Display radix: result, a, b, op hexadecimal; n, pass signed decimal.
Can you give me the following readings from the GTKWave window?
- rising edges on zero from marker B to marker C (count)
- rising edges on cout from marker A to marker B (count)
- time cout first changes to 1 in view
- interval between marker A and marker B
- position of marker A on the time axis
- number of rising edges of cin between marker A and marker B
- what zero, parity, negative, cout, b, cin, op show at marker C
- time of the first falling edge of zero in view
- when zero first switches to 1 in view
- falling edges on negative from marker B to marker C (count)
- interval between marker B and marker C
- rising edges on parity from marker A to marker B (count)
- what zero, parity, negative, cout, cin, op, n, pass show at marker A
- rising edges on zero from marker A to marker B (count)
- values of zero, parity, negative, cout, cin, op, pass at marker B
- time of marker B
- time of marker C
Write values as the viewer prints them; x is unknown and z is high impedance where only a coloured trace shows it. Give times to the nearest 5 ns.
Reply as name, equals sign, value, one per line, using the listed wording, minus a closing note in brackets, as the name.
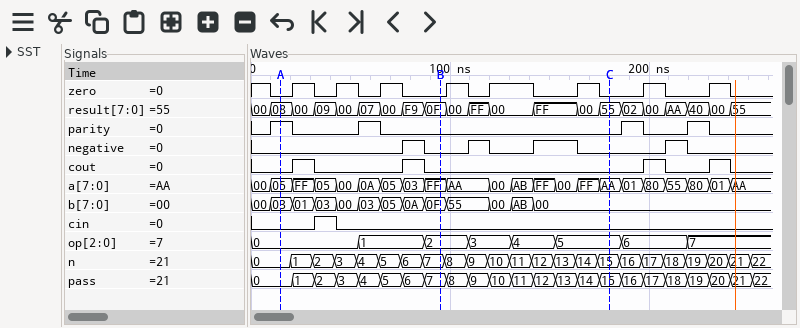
rising edges on zero from marker B to marker C = 3
rising edges on cout from marker A to marker B = 2
time cout first changes to 1 in view = 20 ns
interval between marker A and marker B = 80 ns
position of marker A on the time axis = 15 ns
number of rising edges of cin between marker A and marker B = 1
what zero, parity, negative, cout, b, cin, op show at marker C = zero=0, parity=0, negative=0, cout=0, b=00, cin=0, op=5
time of the first falling edge of zero in view = 10 ns
when zero first switches to 1 in view = 20 ns
falling edges on negative from marker B to marker C = 2
interval between marker B and marker C = 85 ns
rising edges on parity from marker A to marker B = 1
what zero, parity, negative, cout, cin, op, n, pass show at marker A = zero=0, parity=1, negative=0, cout=0, cin=0, op=0, n=0, pass=0
rising edges on zero from marker A to marker B = 3
values of zero, parity, negative, cout, cin, op, pass at marker B = zero=0, parity=0, negative=0, cout=0, cin=0, op=2, pass=7
time of marker B = 95 ns
time of marker C = 180 ns
